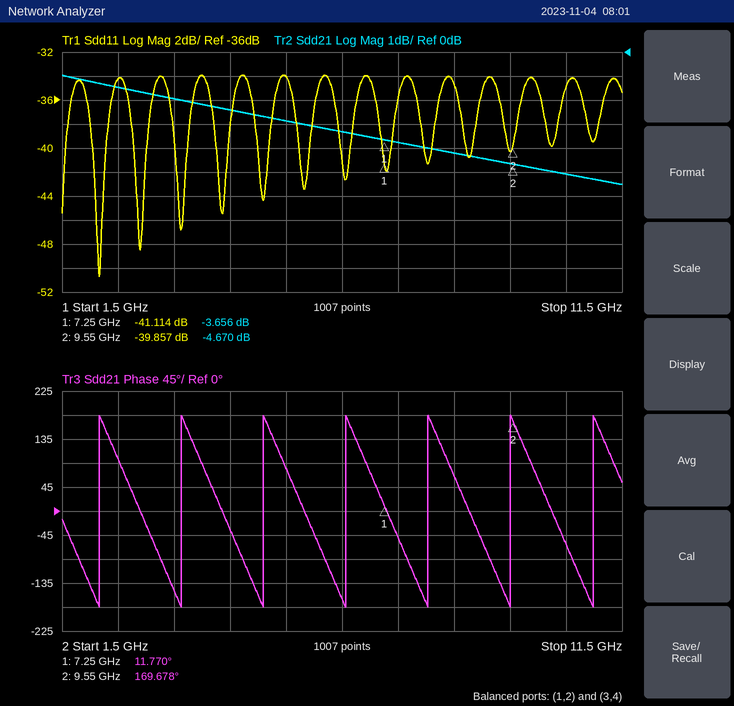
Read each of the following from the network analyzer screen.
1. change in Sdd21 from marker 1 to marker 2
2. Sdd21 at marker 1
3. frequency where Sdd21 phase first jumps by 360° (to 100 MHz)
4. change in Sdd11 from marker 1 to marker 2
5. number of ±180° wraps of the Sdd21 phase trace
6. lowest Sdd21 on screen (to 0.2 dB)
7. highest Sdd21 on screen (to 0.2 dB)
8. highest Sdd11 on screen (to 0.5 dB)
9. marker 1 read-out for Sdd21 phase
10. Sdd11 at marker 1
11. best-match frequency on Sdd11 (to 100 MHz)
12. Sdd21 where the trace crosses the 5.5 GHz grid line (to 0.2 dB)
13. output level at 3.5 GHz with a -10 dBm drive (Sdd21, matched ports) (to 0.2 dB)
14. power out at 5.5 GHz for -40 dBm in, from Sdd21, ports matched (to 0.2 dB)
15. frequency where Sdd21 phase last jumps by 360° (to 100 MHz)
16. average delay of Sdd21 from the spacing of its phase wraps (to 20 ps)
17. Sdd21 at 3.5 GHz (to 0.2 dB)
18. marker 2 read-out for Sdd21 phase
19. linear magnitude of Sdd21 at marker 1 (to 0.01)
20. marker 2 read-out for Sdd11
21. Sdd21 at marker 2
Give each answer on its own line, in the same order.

-1.014 dB
-3.656 dB
2.2 GHz
1.257 dB
7
-5.6 dB
-1.0 dB
-34.0 dB
11.770°
-41.114 dB
2.2 GHz
-2.8 dB
-12.0 dBm
-42.8 dBm
11.0 GHz
680 ps
-2.0 dB
169.678°
0.66
-39.857 dB
-4.670 dB
